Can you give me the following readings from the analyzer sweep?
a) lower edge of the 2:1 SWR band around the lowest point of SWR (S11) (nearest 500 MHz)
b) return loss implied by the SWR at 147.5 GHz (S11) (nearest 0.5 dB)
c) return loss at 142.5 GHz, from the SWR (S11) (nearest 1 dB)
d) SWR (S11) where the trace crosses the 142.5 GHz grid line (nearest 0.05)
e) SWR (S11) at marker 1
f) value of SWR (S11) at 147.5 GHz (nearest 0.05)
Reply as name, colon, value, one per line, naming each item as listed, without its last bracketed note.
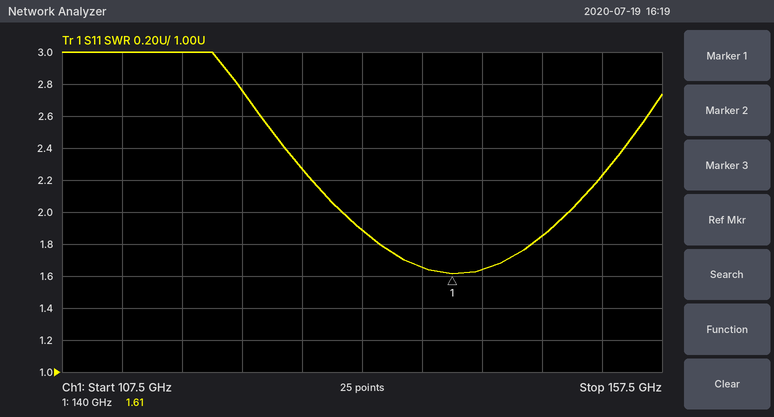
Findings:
lower edge of the 2:1 SWR band around the lowest point of SWR (S11): 131.0 GHz
return loss implied by the SWR at 147.5 GHz (S11): 10.5 dB
return loss at 142.5 GHz, from the SWR (S11): 12 dB
SWR (S11) where the trace crosses the 142.5 GHz grid line: 1.65
SWR (S11) at marker 1: 1.61
value of SWR (S11) at 147.5 GHz: 1.85
